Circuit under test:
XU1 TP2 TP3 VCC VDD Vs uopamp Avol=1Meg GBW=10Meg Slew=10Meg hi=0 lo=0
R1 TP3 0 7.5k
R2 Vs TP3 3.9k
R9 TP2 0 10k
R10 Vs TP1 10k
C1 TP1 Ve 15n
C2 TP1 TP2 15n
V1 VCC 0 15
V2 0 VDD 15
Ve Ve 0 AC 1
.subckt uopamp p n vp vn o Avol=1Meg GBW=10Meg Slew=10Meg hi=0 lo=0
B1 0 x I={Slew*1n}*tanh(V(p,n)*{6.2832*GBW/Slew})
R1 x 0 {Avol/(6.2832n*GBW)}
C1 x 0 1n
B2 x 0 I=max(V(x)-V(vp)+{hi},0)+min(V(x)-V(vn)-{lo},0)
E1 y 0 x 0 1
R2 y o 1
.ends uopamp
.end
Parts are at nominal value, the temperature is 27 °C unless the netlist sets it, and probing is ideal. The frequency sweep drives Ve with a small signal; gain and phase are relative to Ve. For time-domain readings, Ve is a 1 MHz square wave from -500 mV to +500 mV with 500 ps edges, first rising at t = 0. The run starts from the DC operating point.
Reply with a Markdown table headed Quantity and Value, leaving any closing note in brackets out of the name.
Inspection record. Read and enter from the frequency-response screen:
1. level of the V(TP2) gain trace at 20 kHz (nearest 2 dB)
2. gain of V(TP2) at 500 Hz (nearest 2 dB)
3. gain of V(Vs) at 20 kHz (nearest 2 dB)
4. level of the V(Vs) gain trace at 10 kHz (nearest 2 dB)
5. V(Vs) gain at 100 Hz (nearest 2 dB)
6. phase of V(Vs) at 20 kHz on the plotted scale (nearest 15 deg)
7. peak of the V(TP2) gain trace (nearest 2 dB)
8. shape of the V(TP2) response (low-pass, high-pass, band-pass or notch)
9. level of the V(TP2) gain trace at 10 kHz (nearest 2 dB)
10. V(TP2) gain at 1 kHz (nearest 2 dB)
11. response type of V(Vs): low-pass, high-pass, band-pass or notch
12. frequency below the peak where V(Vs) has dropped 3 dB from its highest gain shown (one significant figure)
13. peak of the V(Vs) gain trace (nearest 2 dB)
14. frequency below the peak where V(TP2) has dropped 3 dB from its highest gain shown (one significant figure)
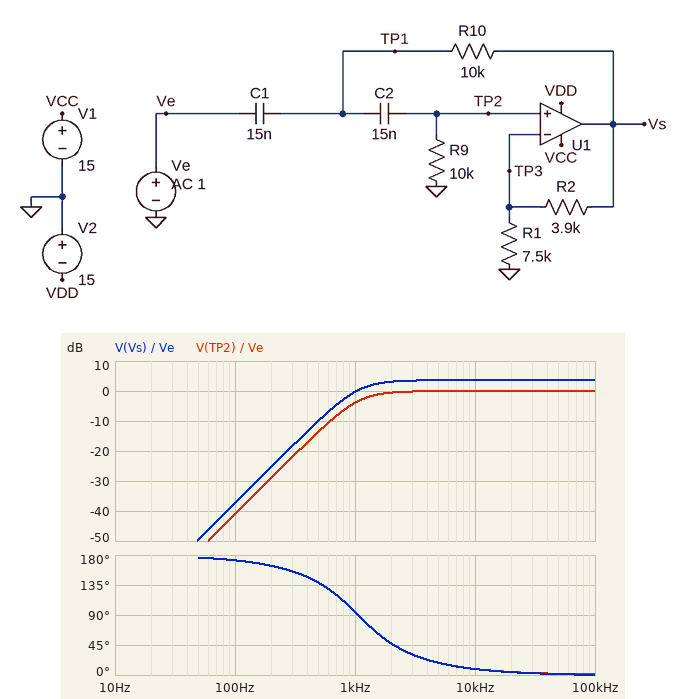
| Quantity | Value |
|---|---|
| level of the V(TP2) gain trace at 20 kHz | 0 dB |
| gain of V(TP2) at 500 Hz | -14 dB |
| gain of V(Vs) at 20 kHz | 4 dB |
| level of the V(Vs) gain trace at 10 kHz | 4 dB |
| V(Vs) gain at 100 Hz | -38 dB |
| phase of V(Vs) at 20 kHz on the plotted scale | 0 deg |
| peak of the V(TP2) gain trace | 0 dB |
| shape of the V(TP2) response | high-pass |
| level of the V(TP2) gain trace at 10 kHz | 0 dB |
| V(TP2) gain at 1 kHz | -4 dB |
| response type of V(Vs): low-pass, high-pass, band-pass or notch | high-pass |
| frequency below the peak where V(Vs) has dropped 3 dB from its highest gain shown | 1 kHz |
| peak of the V(Vs) gain trace | 4 dB |
| frequency below the peak where V(TP2) has dropped 3 dB from its highest gain shown | 1 kHz |
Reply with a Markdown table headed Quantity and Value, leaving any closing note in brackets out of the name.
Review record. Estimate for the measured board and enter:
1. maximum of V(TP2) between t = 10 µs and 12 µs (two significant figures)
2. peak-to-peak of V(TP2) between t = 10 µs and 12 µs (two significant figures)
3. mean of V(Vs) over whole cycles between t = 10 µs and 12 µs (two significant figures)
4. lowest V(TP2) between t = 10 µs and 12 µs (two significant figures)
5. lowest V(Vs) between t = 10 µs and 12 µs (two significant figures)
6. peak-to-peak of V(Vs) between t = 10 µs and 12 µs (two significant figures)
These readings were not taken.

| Quantity | Value |
|---|---|
| maximum of V(TP2) between t = 10 µs and 12 µs | 950 mV |
| peak-to-peak of V(TP2) between t = 10 µs and 12 µs | 1.0 V |
| mean of V(Vs) over whole cycles between t = 10 µs and 12 µs | 680 mV |
| lowest V(TP2) between t = 10 µs and 12 µs | -58 mV |
| lowest V(Vs) between t = 10 µs and 12 µs | -87 mV |
| peak-to-peak of V(Vs) between t = 10 µs and 12 µs | 1.5 V |
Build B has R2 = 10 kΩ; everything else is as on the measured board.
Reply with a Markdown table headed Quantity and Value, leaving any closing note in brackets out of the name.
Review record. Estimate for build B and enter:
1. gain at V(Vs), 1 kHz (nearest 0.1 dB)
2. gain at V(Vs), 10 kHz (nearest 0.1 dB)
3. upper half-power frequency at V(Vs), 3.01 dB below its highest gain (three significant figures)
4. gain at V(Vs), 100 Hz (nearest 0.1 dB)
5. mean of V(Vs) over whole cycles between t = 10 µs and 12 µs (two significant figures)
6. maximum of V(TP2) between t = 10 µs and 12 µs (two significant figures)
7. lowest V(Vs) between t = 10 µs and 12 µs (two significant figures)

| Quantity | Value |
|---|---|
| gain at V(Vs), 1 kHz | 10.2 dB |
| gain at V(Vs), 10 kHz | 7.4 dB |
| upper half-power frequency at V(Vs), 3.01 dB below its highest gain | 2.74 kHz |
| gain at V(Vs), 100 Hz | -33.6 dB |
| mean of V(Vs) over whole cycles between t = 10 µs and 12 µs | 1.1 V |
| maximum of V(TP2) between t = 10 µs and 12 µs | 980 mV |
| lowest V(Vs) between t = 10 µs and 12 µs | -64 mV |
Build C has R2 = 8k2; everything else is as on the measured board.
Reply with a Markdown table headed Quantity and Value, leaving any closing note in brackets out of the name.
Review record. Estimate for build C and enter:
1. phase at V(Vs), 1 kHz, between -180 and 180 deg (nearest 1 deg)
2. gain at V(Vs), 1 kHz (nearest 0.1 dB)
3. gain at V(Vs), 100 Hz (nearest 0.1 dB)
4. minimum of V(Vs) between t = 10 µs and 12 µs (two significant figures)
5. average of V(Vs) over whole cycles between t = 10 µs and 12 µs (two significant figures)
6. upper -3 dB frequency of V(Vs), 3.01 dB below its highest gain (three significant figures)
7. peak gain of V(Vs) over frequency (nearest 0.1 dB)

| Quantity | Value |
|---|---|
| phase at V(Vs), 1 kHz, between -180 and 180 deg | 97 deg |
| gain at V(Vs), 1 kHz | 6.7 dB |
| gain at V(Vs), 100 Hz | -34.6 dB |
| minimum of V(Vs) between t = 10 µs and 12 µs | -76 mV |
| average of V(Vs) over whole cycles between t = 10 µs and 12 µs | 980 mV |
| upper -3 dB frequency of V(Vs), 3.01 dB below its highest gain | 2.64 MHz |
| peak gain of V(Vs) over frequency | 8.3 dB |
